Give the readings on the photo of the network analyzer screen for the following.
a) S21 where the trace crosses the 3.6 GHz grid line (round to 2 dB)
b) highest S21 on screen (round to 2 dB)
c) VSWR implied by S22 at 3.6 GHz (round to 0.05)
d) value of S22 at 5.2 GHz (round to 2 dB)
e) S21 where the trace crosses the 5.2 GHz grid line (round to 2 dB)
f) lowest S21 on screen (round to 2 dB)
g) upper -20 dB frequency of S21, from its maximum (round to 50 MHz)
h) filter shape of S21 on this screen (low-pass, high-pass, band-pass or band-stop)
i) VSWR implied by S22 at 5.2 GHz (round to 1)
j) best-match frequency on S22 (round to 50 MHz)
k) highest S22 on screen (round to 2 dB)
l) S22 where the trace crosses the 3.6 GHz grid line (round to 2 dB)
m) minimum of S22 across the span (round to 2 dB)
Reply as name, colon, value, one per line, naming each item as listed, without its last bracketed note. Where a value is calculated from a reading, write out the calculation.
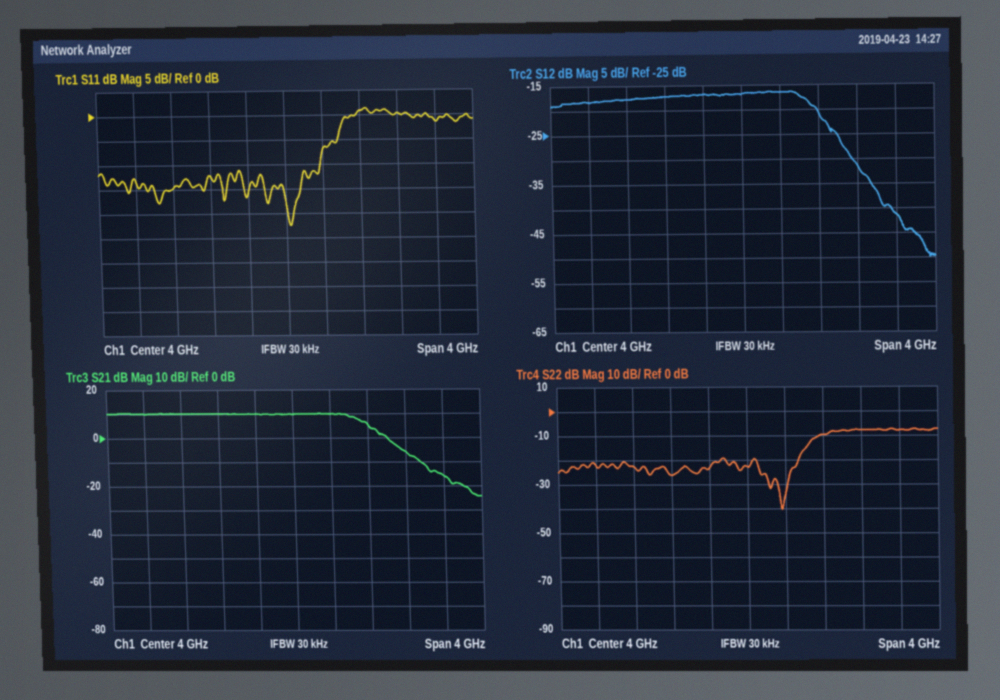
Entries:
S21 where the trace crosses the 3.6 GHz grid line: 10 dB
highest S21 on screen: 10 dB
VSWR implied by S22 at 3.6 GHz: |Γ| = 10^(-24/20) = 0.0631; VSWR = (1 + 0.0631)/(1 − 0.0631) ≈ 1.13, so 1.15 to the nearest 0.05
value of S22 at 5.2 GHz: -8 dB
S21 where the trace crosses the 5.2 GHz grid line: -6 dB
lowest S21 on screen: -24 dB
upper -20 dB frequency of S21, from its maximum: 5.35 GHz
filter shape of S21 on this screen: low-pass
VSWR implied by S22 at 5.2 GHz: |Γ| = 10^(-8/20) = 0.3981; VSWR = (1 + 0.3981)/(1 − 0.3981) ≈ 2
best-match frequency on S22: 4.35 GHz
highest S22 on screen: -8 dB
S22 where the trace crosses the 3.6 GHz grid line: -24 dB
minimum of S22 across the span: -40 dB
